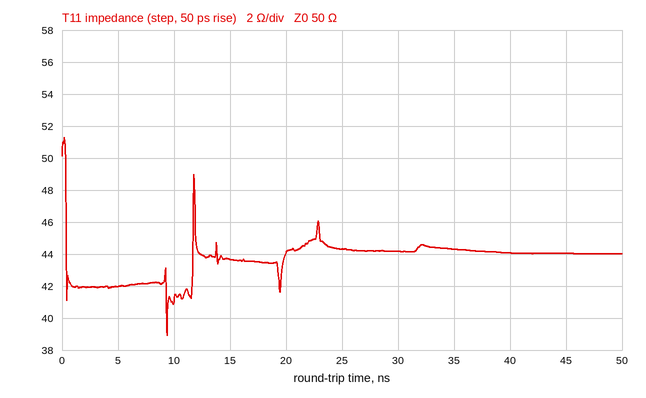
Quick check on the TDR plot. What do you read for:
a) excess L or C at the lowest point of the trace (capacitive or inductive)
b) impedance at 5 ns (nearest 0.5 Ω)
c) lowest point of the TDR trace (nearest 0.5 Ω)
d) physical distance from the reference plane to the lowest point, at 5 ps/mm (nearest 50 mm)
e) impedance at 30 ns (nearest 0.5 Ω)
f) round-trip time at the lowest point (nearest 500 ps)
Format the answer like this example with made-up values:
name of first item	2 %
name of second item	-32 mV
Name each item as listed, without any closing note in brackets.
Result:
excess L or C at the lowest point of the trace	capacitive
impedance at 5 ns	42.0 Ω
lowest point of the TDR trace	39.0 Ω
physical distance from the reference plane to the lowest point, at 5 ps/mm	950 mm
impedance at 30 ns	44.0 Ω
round-trip time at the lowest point	9.5 ns
